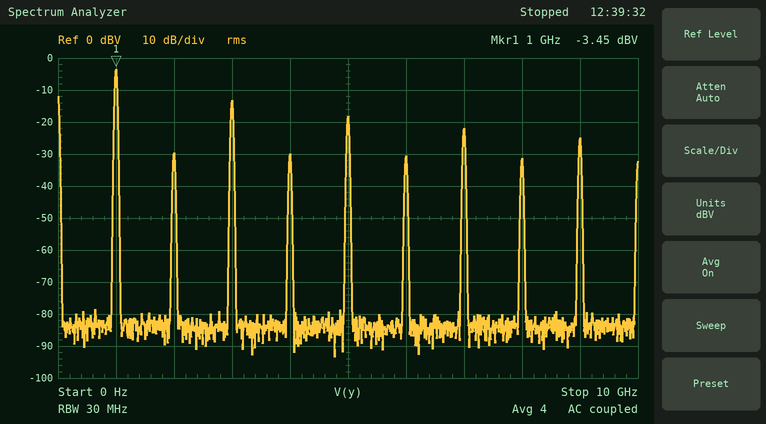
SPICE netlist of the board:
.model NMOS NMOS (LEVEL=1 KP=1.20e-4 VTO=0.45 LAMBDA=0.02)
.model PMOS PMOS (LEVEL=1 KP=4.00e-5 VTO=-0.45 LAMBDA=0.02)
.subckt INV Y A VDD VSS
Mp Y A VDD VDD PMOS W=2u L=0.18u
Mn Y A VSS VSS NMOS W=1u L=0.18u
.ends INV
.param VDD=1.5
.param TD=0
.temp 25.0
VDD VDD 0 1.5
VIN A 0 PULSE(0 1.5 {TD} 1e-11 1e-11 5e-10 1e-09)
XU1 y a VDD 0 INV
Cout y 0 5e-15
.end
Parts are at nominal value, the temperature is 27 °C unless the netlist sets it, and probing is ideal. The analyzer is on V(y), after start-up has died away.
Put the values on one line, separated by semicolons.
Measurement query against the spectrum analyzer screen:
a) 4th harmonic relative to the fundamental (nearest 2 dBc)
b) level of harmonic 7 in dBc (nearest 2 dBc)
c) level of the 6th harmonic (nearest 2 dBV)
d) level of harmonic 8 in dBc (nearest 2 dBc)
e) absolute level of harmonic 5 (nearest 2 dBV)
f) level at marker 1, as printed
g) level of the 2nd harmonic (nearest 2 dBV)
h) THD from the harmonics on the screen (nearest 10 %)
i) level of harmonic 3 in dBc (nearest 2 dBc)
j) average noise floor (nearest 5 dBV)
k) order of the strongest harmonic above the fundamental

-26 dBc; -18 dBc; -30 dBV; -28 dBc; -18 dBV; -3.45 dBV; -30 dBV; 40 %; -10 dBc; -85 dBV; 3
